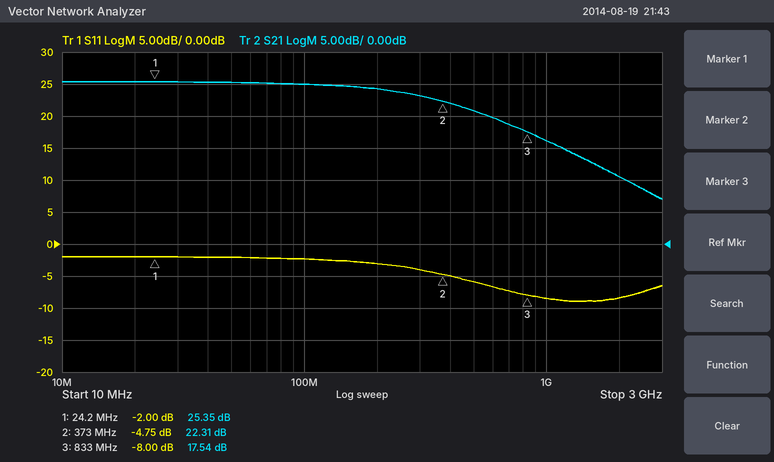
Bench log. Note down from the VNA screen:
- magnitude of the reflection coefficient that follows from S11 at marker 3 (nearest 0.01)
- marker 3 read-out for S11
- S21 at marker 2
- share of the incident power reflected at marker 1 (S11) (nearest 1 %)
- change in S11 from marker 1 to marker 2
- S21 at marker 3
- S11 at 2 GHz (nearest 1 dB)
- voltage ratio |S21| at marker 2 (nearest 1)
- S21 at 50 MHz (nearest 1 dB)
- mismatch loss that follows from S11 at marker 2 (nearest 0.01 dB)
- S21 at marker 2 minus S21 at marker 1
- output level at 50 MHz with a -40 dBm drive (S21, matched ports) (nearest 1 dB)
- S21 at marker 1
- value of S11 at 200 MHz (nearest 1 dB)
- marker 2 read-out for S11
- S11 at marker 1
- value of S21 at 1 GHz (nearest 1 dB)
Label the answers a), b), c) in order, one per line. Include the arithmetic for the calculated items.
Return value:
a) 10^(-8/20) ≈ 0.40
b) -8.00 dB
c) 22.31 dB
d) 10^(-2/10) ≈ 63 %
e) -4.75 − (-2) = -2.75 dB
f) 17.54 dB
g) -8 dB
h) 10^(22.31/20) ≈ 13
i) 25 dB
j) −10 log10(1 − 10^(-4.75/10)) ≈ 1.77 dB
k) 22.31 − (25.35) = -3.04 dB
l) -40 dBm + (25 dB) = -15 dBm
m) 25.35 dB
n) -3 dB
o) -4.75 dB
p) -2.00 dB
q) 16 dB
